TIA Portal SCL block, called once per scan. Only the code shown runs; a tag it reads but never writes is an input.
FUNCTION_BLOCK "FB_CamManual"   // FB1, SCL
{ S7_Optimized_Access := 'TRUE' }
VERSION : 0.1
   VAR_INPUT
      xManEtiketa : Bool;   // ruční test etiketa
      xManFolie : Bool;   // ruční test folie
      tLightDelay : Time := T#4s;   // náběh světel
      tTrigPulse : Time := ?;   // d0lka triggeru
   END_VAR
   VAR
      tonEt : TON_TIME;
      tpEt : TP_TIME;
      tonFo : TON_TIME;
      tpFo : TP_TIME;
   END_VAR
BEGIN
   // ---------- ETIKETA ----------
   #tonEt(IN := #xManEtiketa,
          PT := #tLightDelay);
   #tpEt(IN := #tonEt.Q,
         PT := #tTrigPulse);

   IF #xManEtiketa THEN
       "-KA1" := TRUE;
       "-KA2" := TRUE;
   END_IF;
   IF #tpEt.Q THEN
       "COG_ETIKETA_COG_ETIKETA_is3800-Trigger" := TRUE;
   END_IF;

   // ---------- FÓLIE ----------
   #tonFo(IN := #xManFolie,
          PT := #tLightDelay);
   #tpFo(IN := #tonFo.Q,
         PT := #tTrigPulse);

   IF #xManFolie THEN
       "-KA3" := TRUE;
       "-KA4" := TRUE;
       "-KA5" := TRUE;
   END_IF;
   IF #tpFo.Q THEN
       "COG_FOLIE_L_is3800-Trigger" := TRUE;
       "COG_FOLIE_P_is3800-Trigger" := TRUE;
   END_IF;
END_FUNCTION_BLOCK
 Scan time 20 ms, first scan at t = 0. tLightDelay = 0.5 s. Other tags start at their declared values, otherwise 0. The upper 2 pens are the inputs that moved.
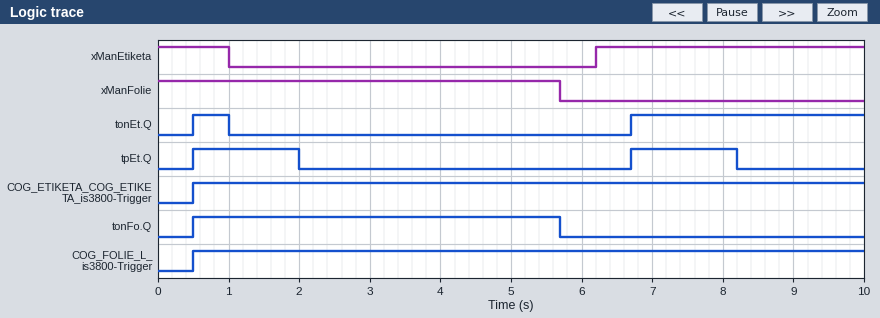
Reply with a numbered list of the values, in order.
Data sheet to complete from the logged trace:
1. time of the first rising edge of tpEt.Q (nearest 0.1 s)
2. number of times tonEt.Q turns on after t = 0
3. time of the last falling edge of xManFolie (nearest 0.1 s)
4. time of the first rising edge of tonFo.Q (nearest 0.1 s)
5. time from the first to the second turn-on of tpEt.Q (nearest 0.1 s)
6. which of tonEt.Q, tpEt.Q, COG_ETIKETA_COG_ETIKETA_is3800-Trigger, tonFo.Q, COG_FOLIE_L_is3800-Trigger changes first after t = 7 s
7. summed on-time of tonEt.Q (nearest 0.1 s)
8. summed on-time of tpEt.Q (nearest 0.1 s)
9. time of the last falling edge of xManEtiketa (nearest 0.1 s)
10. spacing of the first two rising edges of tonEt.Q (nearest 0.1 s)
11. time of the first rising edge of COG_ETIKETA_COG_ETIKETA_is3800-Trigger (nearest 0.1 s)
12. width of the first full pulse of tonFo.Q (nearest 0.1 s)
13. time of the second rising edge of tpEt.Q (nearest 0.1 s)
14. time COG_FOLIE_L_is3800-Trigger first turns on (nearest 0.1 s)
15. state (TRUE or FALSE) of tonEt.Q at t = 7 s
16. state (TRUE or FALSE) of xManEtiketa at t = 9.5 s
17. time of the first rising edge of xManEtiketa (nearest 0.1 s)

1. 0.5 s
2. 2
3. 5.7 s
4. 0.5 s
5. 6.2 s
6. tpEt.Q
7. 3.8 s
8. 3.0 s
9. 1.0 s
10. 6.2 s
11. 0.5 s
12. 5.2 s
13. 6.7 s
14. 0.5 s
15. TRUE
16. TRUE
17. 6.2 s
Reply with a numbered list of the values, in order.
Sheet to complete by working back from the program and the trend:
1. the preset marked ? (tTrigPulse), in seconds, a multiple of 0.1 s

1. 1.5 s
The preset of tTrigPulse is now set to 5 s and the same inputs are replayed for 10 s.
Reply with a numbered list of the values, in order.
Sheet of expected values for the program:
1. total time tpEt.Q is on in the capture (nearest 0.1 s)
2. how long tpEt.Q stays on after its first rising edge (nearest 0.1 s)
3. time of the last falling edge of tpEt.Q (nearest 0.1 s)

1. 8.3 s
2. 5.0 s
3. 5.5 s
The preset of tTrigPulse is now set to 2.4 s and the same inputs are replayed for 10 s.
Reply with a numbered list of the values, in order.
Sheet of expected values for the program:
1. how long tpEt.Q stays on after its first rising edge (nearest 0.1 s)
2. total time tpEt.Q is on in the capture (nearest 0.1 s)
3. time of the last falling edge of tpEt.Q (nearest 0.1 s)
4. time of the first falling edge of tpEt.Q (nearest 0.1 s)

1. 2.4 s
2. 4.8 s
3. 9.1 s
4. 2.9 s
